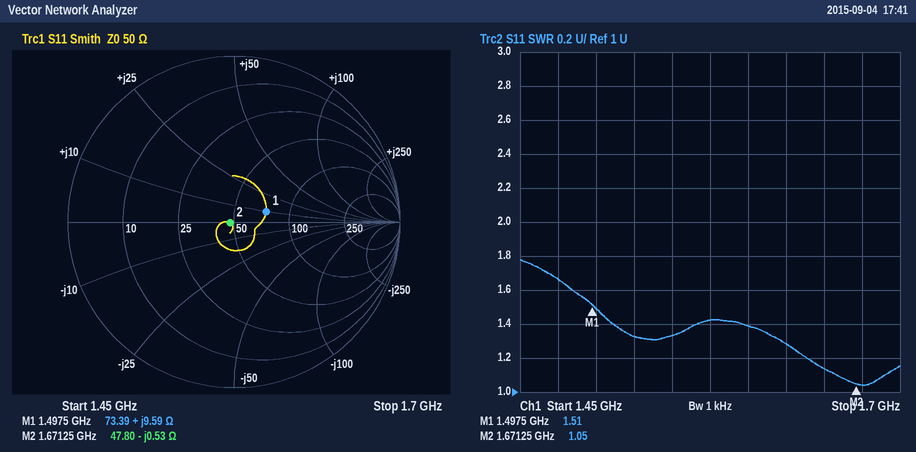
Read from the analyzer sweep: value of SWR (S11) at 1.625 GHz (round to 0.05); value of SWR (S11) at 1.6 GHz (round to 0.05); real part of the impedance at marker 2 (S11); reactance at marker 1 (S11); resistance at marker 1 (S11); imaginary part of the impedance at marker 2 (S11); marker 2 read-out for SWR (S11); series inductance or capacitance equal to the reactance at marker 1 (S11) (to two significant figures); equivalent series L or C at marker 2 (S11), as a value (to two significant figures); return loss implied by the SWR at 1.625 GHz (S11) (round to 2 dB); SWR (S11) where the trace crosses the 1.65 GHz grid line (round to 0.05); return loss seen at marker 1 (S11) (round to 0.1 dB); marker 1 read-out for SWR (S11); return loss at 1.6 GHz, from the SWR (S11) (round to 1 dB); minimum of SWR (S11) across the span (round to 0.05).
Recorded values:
1.30
1.40
47.80 Ω
+9.59 Ω
73.39 Ω
-0.53 Ω
1.05
1.0 nH
180 pF
18 dB
1.15
13.8 dB
1.51
16 dB
1.05
